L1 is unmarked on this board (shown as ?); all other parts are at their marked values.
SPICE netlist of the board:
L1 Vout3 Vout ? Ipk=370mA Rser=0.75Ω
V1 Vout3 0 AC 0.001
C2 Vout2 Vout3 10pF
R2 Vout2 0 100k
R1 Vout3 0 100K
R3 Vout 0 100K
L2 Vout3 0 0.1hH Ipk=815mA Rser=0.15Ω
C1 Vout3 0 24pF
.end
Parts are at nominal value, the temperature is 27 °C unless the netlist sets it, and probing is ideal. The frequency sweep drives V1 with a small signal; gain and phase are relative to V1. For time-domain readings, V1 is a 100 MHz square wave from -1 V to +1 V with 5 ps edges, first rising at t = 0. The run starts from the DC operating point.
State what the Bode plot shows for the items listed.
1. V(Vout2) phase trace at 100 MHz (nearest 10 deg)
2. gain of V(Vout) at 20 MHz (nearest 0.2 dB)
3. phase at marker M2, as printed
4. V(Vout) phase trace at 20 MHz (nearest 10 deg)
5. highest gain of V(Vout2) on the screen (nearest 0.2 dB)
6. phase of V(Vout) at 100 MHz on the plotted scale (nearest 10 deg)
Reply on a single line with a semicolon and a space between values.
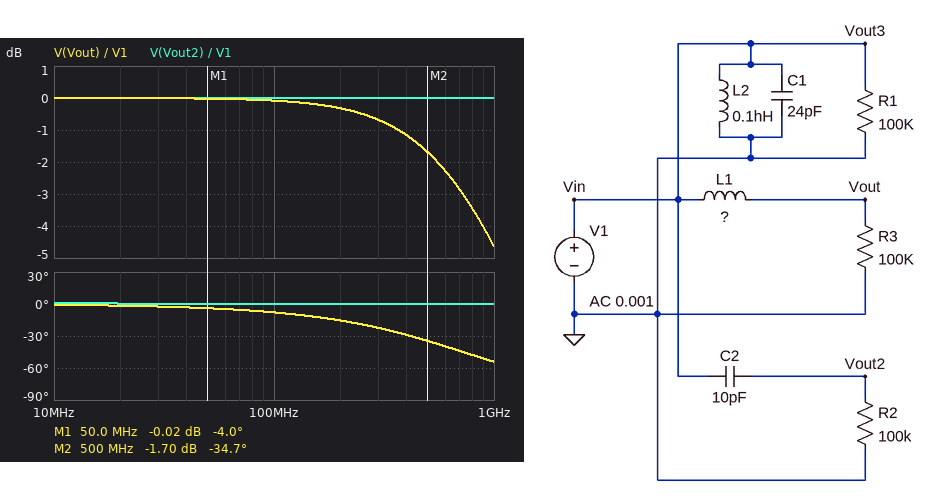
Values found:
0 deg; 0 dB; -34.7 deg; 0 deg; 0 dB; -10 deg
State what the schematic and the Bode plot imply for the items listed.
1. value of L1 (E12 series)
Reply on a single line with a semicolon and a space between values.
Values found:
22 µH
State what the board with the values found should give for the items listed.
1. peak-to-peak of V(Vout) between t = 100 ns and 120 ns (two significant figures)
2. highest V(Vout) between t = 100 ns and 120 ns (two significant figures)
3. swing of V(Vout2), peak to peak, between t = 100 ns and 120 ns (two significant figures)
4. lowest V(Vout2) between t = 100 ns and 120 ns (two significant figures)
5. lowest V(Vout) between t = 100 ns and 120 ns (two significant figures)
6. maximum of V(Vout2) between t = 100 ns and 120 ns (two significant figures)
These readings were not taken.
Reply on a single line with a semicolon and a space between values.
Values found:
2.0 V; 1.0 V; 2.0 V; -110 mV; -1.0 V; 1.9 V
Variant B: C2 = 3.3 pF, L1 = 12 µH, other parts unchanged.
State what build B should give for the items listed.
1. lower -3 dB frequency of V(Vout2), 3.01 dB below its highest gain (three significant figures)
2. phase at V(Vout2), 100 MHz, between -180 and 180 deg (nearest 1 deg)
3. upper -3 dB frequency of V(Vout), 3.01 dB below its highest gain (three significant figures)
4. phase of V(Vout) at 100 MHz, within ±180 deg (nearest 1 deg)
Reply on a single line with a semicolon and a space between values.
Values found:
482 kHz; 0 deg; 1.33 GHz; -4 deg
